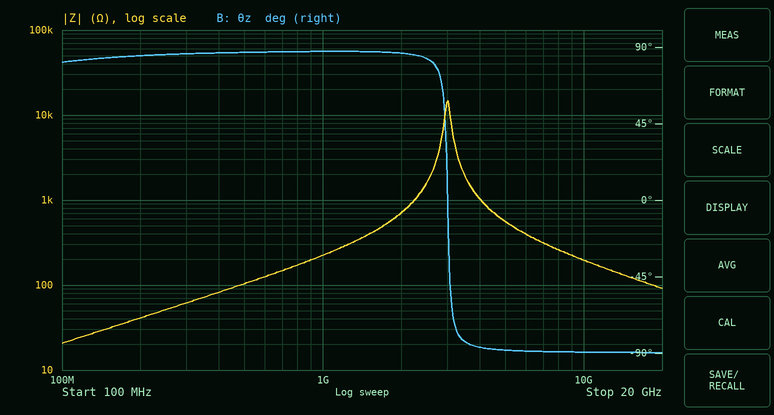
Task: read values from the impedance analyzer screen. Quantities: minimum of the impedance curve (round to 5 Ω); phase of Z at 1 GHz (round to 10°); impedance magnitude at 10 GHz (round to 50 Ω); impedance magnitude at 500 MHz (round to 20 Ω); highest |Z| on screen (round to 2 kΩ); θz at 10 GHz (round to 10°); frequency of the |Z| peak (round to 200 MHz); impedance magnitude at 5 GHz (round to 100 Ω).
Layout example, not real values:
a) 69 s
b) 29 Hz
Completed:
a) 20 Ω
b) 90°
c) 200 Ω
d) 100 Ω
e) 14 kΩ
f) -90°
g) 3.0 GHz
h) 600 Ω
